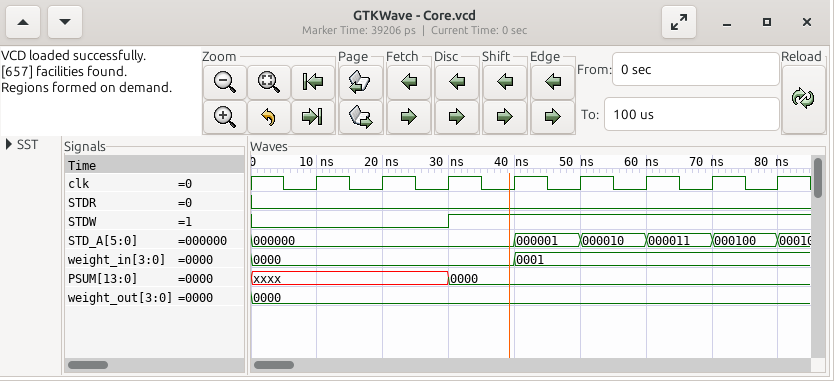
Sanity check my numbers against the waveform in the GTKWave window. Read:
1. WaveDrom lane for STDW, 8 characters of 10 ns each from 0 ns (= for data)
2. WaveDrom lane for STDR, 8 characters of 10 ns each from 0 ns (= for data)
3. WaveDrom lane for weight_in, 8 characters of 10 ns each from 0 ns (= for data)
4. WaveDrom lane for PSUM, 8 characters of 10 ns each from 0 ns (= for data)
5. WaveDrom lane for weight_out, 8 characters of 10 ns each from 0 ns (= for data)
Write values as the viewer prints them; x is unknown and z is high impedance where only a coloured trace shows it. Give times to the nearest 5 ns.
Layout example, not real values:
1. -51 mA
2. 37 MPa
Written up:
1. {name: 'STDW', wave: '0..1....'}
2. {name: 'STDR', wave: '0.......'}
3. {name: 'weight_in', wave: '=...=...', data: '0000 0001'}
4. {name: 'PSUM', wave: 'x..=....', data: '0000'}
5. {name: 'weight_out', wave: '=.......', data: '0000'}
